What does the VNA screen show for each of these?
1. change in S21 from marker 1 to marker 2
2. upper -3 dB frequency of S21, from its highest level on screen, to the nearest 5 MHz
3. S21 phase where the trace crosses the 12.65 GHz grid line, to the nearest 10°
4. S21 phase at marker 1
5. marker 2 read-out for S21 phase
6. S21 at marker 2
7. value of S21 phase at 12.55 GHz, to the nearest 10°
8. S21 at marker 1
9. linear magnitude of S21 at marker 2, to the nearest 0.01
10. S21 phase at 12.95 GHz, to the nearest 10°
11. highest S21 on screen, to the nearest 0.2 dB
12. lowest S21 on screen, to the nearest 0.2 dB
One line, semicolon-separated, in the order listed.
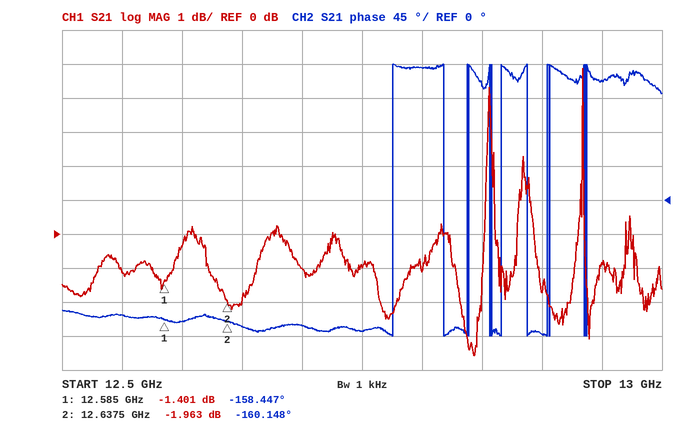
-0.562 dB; 12.935 GHz; -170°; -158.447°; -160.148°; -1.963 dB; -150°; -1.401 dB; 0.80; 160°; 4.8 dB; -3.6 dB
